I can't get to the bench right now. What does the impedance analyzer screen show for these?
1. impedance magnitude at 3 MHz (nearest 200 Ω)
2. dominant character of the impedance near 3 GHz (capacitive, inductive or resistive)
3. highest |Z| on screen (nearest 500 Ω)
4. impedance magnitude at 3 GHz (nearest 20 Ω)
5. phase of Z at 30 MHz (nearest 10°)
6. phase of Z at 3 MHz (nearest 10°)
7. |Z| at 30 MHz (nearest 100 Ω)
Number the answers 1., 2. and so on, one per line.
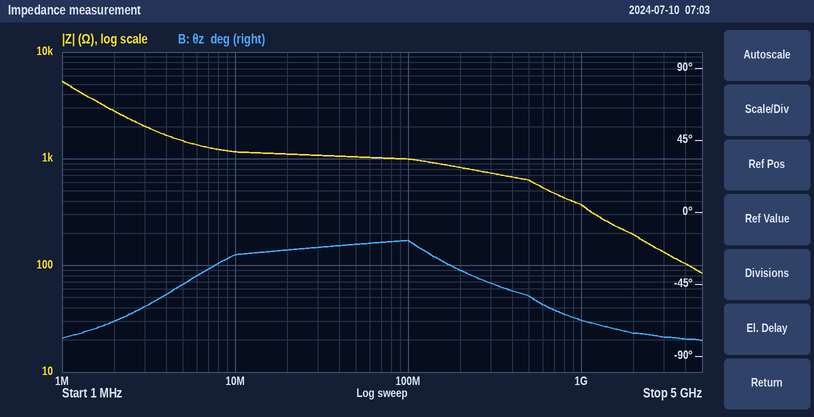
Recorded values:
1. 2.0 kΩ
2. capacitive
3. 5.5 kΩ
4. 140 Ω
5. -20°
6. -60°
7. 1.1 kΩ
